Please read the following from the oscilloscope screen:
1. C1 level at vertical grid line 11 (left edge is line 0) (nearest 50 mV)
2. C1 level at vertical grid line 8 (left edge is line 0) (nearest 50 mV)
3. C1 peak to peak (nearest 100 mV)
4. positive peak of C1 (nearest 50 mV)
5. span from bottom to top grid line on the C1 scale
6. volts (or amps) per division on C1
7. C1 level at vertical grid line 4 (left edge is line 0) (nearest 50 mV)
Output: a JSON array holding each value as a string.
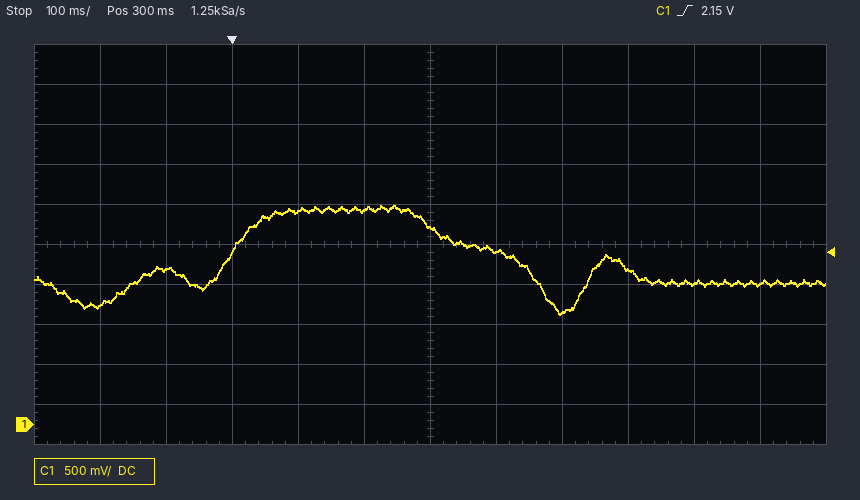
["1.75 V", "1.40 V", "1.40 V", "2.75 V", "5 V", "500 mV", "2.65 V"]
